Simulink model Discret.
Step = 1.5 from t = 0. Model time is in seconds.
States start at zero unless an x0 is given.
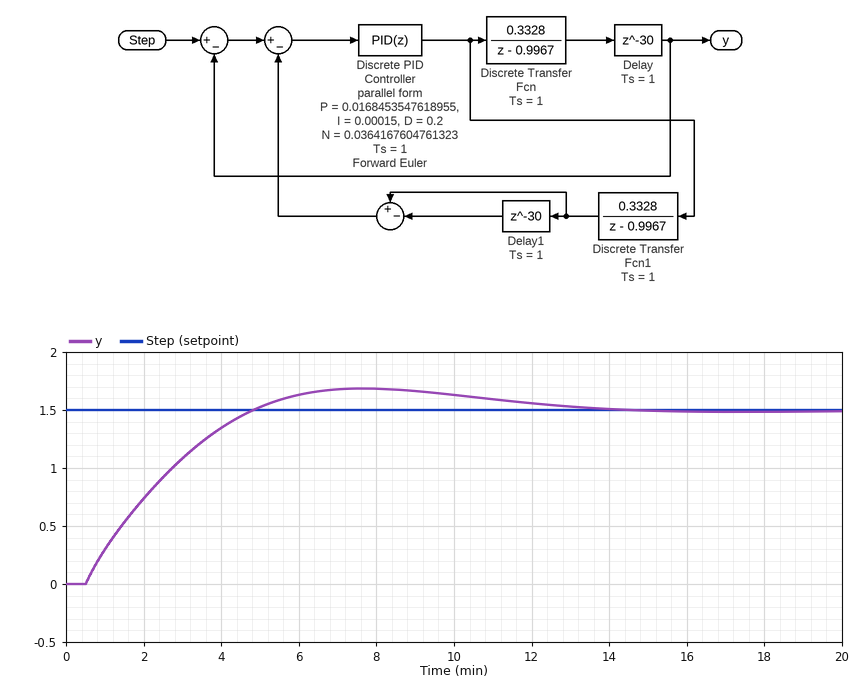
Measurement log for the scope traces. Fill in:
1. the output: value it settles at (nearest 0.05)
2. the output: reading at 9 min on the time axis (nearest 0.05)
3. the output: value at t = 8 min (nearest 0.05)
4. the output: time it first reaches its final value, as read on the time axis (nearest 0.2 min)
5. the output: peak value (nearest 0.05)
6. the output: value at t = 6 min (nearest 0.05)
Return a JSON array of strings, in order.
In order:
["1.50", "1.65", "1.70", "4.8 min", "1.70", "1.65"]
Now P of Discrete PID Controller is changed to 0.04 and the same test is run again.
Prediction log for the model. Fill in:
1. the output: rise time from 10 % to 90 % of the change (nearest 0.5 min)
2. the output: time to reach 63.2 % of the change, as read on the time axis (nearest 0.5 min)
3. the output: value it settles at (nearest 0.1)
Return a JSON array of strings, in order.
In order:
["2.5 min", "1.5 min", "1.5"]
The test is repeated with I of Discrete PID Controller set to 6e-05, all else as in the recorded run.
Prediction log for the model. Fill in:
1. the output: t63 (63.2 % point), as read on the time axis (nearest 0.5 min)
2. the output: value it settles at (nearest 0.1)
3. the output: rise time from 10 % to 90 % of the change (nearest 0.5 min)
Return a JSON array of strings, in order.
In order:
["3.5 min", "1.5", "6.5 min"]
